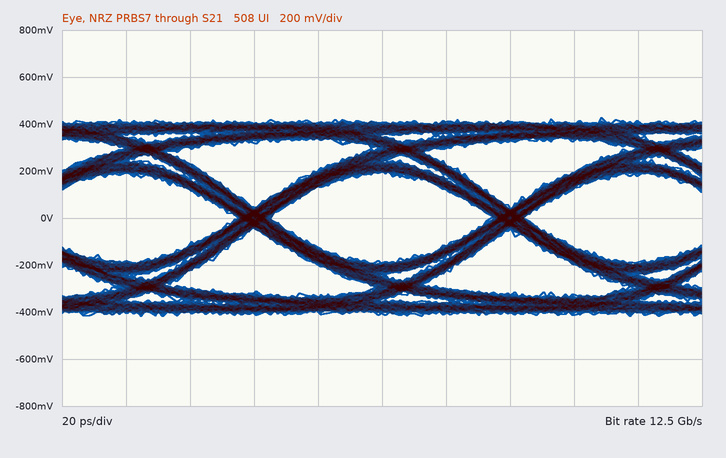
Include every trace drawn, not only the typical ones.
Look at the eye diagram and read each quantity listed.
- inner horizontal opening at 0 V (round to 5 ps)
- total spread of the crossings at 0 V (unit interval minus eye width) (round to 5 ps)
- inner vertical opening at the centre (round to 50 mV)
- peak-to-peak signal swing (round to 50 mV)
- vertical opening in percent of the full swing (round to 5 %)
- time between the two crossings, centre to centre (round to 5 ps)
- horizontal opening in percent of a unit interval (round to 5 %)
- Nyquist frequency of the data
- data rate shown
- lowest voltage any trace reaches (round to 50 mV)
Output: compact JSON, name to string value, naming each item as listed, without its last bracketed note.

{"inner horizontal opening at 0 V": "70 ps", "total spread of the crossings at 0 V (unit interval minus eye width)": "10 ps", "inner vertical opening at the centre": "400 mV", "peak-to-peak signal swing": "850 mV", "vertical opening in percent of the full swing": "45 %", "time between the two crossings, centre to centre": "80 ps", "horizontal opening in percent of a unit interval": "85 %", "Nyquist frequency of the data": "6.25 GHz", "data rate shown": "12.5 Gb/s", "lowest voltage any trace reaches": "-400 mV"}
